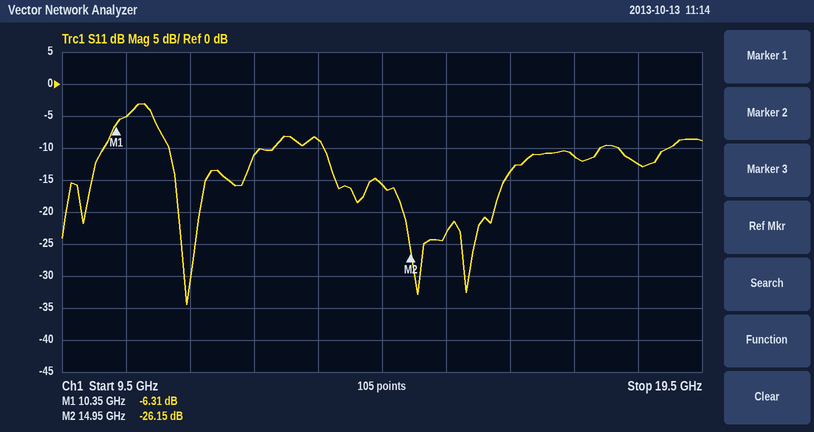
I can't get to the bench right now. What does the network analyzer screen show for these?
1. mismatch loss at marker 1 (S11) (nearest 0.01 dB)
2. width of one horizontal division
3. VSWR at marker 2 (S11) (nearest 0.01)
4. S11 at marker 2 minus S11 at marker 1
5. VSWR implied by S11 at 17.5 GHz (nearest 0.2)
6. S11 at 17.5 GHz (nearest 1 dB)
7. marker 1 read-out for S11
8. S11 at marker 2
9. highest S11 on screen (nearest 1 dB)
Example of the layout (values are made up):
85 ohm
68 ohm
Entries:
1.16 dB
1 GHz
1.10
-19.84 dB
1.8
-11 dB
-6.31 dB
-26.15 dB
-3 dB
